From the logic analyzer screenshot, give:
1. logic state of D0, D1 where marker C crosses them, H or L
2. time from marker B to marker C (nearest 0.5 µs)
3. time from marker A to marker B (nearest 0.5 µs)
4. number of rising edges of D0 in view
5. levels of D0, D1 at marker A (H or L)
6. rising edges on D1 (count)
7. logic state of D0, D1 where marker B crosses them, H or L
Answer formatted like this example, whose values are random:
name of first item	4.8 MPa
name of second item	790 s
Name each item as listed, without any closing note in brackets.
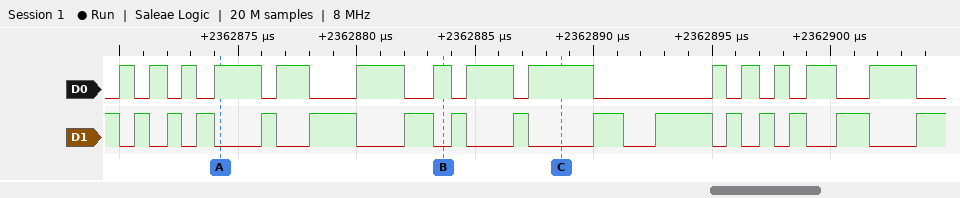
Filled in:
logic state of D0, D1 where marker C crosses them, H or L	D0=H, D1=L
time from marker B to marker C	5 µs
time from marker A to marker B	9.5 µs
number of rising edges of D0 in view	14
levels of D0, D1 at marker A	D0=H, D1=L
rising edges on D1	15
logic state of D0, D1 where marker B crosses them, H or L	D0=H, D1=L
